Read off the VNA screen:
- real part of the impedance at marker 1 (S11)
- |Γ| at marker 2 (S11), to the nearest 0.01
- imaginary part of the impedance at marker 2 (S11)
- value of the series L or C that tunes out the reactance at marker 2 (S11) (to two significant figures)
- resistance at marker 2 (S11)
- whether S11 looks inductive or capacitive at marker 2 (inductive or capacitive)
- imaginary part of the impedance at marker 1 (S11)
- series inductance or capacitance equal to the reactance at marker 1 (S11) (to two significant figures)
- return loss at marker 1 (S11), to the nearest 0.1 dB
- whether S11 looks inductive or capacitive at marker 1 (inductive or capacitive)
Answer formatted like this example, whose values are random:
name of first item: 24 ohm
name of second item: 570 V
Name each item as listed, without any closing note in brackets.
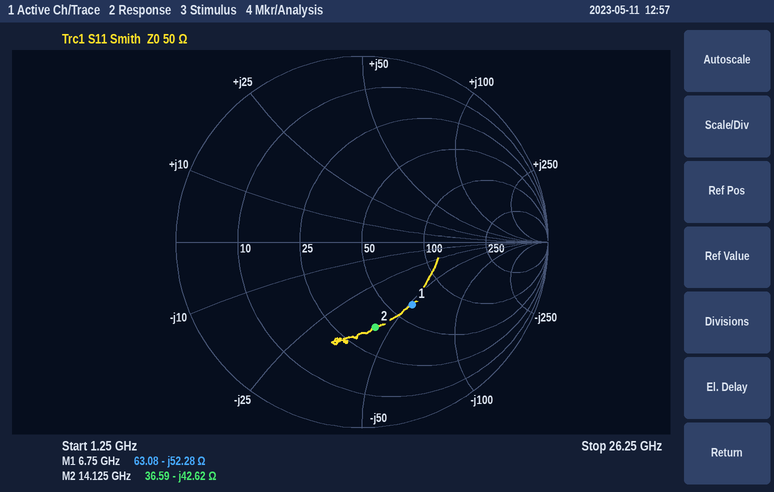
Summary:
real part of the impedance at marker 1: 63.08 Ω
|Γ| at marker 2 (S11), to the nearest 0.01: 0.46
imaginary part of the impedance at marker 2: -42.62 Ω
value of the series L or C that tunes out the reactance at marker 2 (S11): 480 pH
resistance at marker 2: 36.59 Ω
whether S11 looks inductive or capacitive at marker 2: capacitive
imaginary part of the impedance at marker 1: -52.28 Ω
series inductance or capacitance equal to the reactance at marker 1 (S11): 450 fF
return loss at marker 1 (S11), to the nearest 0.1 dB: 7.3 dB
whether S11 looks inductive or capacitive at marker 1: capacitive
